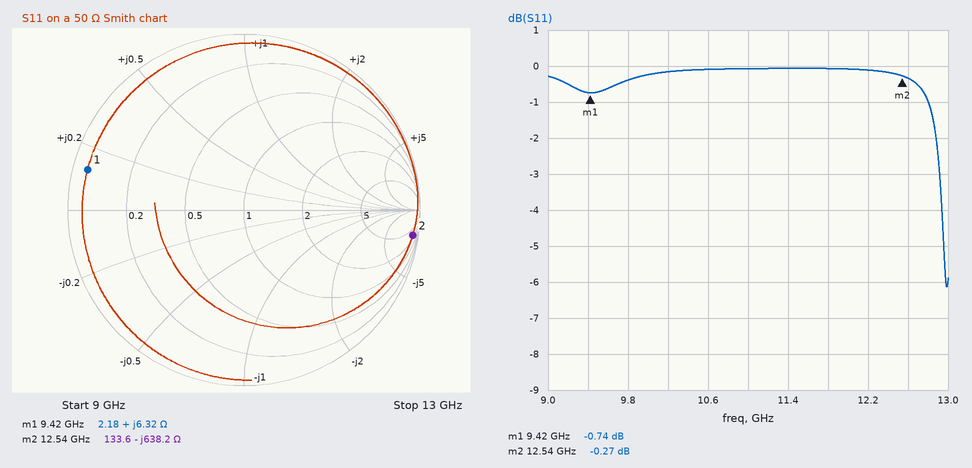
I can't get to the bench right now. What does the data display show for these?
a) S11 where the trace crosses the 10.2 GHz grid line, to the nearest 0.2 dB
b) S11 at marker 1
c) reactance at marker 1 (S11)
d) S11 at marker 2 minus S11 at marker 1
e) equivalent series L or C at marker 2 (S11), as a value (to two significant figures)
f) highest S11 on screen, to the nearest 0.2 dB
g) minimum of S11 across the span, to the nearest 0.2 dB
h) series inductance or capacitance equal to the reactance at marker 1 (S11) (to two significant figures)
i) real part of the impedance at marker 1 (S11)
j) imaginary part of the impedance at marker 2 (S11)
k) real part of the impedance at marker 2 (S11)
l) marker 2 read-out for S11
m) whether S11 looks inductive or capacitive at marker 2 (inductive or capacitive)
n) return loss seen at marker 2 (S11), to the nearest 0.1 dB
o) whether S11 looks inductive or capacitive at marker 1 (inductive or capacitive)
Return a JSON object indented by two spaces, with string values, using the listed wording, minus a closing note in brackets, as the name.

{
  "S11 where the trace crosses the 10.2 GHz grid line, to the nearest 0.2 dB": "-0.2 dB",
  "S11 at marker 1": "-0.74 dB",
  "reactance at marker 1": "+6.32 Ω",
  "S11 at marker 2 minus S11 at marker 1": "0.47 dB",
  "equivalent series L or C at marker 2 (S11), as a value": "20 fF",
  "highest S11 on screen, to the nearest 0.2 dB": "0.0 dB",
  "minimum of S11 across the span, to the nearest 0.2 dB": "-6.2 dB",
  "series inductance or capacitance equal to the reactance at marker 1 (S11)": "110 pH",
  "real part of the impedance at marker 1": "2.18 Ω",
  "imaginary part of the impedance at marker 2": "-638.2 Ω",
  "real part of the impedance at marker 2": "133.6 Ω",
  "marker 2 read-out for S11": "-0.27 dB",
  "whether S11 looks inductive or capacitive at marker 2": "capacitive",
  "return loss seen at marker 2 (S11), to the nearest 0.1 dB": "0.3 dB",
  "whether S11 looks inductive or capacitive at marker 1": "inductive"
}
